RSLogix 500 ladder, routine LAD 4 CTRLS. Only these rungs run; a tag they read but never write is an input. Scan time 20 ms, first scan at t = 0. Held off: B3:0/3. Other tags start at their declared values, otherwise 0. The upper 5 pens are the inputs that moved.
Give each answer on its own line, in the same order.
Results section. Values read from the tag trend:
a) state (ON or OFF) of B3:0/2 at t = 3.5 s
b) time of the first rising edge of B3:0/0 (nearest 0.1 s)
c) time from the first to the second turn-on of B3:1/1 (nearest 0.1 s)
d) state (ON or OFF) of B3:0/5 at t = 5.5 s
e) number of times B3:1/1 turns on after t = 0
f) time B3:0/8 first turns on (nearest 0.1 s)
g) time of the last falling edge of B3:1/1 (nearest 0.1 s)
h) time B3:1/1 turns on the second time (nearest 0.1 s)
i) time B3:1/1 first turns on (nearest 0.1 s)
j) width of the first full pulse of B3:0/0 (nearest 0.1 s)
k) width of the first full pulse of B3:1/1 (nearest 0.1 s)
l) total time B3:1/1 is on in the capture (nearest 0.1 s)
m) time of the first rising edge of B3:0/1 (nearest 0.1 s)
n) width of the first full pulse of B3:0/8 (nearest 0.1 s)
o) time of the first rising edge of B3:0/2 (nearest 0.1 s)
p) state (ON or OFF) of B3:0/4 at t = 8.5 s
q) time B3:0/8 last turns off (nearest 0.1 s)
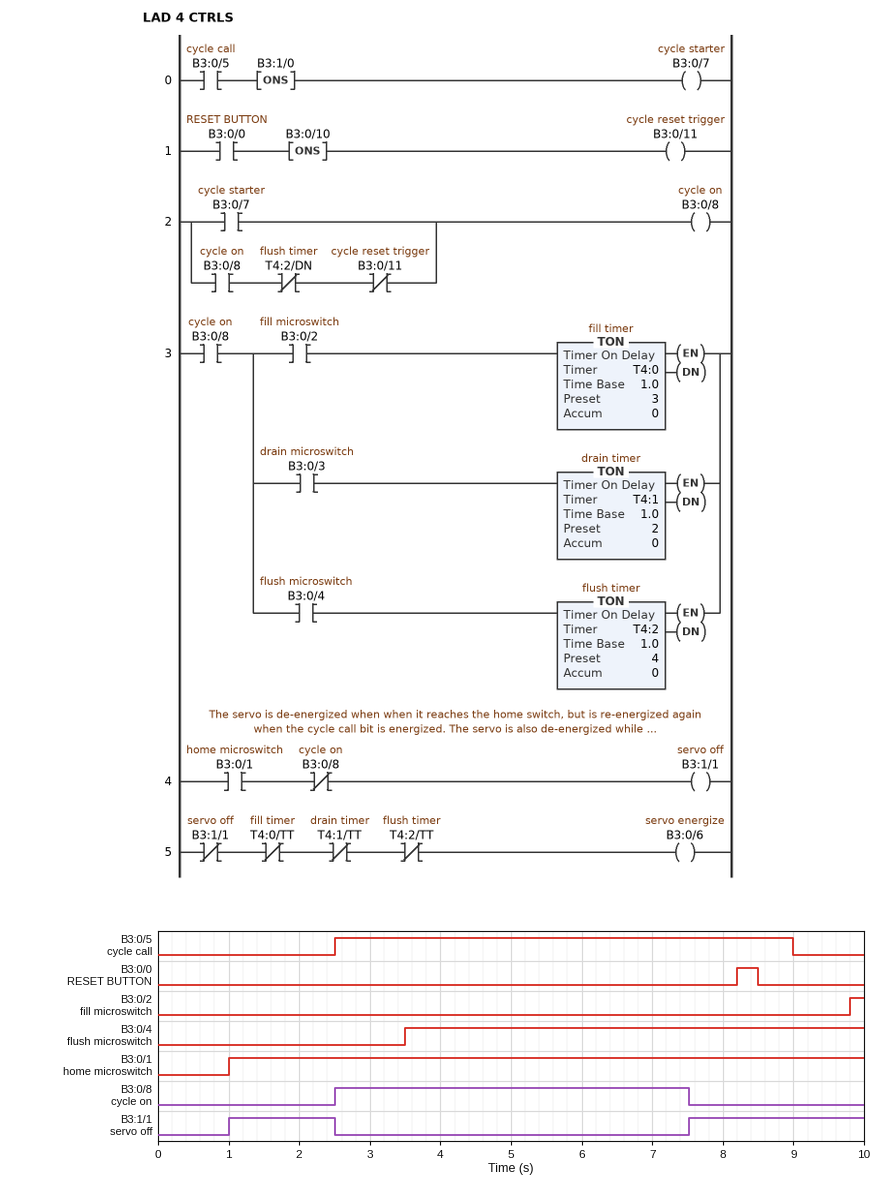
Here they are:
OFF
8.2 s
6.5 s
ON
2
2.5 s
2.5 s
7.5 s
1.0 s
0.3 s
1.5 s
4.0 s
1.0 s
5.0 s
9.8 s
ON
7.5 s
